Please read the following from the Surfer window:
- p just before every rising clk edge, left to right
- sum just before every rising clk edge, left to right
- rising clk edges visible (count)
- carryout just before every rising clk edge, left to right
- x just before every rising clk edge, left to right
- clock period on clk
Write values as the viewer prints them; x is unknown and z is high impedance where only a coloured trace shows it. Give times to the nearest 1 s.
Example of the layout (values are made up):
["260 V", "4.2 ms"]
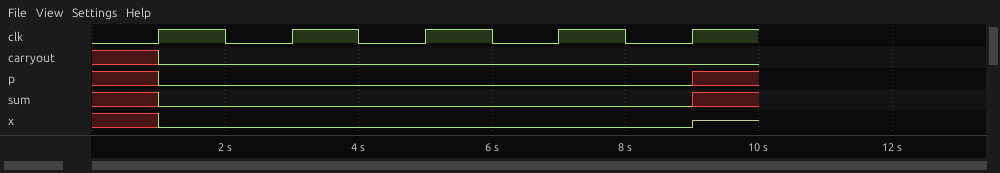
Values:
["x 0 0 0 0", "x 0 0 0 0", "5", "x 0 0 0 0", "x 0 0 0 0", "2 s"]
